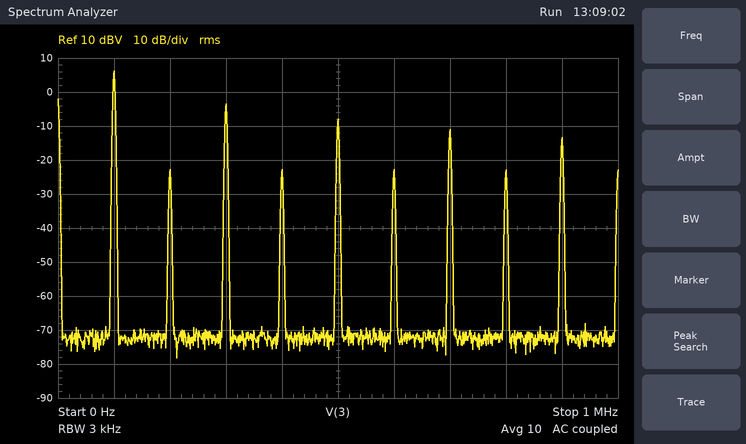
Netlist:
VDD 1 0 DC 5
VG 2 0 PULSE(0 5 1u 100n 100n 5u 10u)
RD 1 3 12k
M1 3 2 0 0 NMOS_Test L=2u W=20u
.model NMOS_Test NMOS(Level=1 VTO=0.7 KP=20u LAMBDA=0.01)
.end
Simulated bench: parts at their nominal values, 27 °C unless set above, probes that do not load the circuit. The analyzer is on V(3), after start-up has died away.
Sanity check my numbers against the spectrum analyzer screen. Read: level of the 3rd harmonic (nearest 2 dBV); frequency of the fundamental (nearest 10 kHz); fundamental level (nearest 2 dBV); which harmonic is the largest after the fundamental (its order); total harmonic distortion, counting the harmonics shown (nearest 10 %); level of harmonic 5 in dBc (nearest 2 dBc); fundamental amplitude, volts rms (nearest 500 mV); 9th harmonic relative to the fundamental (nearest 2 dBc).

-4 dBV
100 kHz
6 dBV
3
40 %
-14 dBc
2.0 V
-20 dBc
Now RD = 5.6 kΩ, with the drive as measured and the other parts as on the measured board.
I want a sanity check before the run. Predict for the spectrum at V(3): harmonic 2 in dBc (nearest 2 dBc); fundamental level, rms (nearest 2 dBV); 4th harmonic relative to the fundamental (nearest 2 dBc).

-30 dBc
6 dBV
-30 dBc
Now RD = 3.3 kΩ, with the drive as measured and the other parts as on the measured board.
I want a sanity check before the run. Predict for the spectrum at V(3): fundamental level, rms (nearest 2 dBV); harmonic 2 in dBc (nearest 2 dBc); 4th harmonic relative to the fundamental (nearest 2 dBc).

4 dBV
-32 dBc
-32 dBc
